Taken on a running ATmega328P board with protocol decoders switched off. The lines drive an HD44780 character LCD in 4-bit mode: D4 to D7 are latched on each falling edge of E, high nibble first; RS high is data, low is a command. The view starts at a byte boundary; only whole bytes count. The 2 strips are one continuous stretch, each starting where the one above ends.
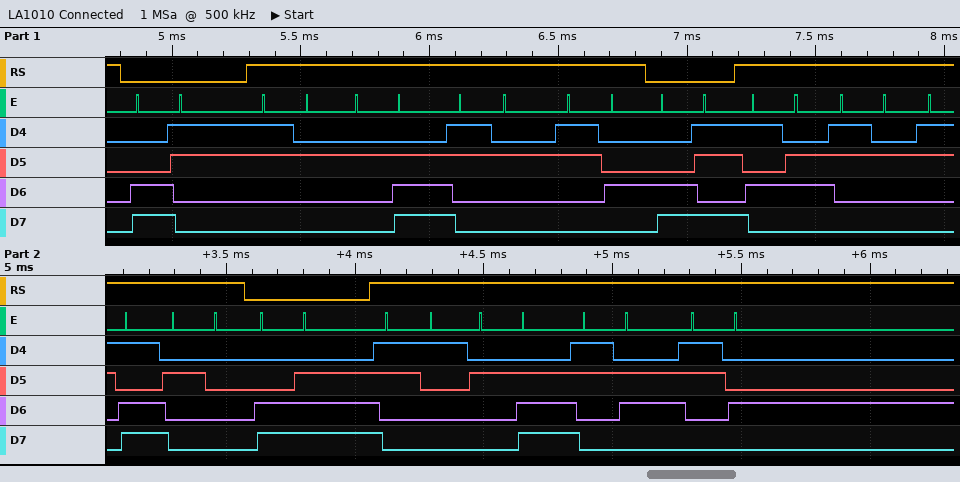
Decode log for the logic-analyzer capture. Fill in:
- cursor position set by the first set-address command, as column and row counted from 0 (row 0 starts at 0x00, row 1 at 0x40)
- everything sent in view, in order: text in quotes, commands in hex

column 3, row 1
0xC3 "2.24" 0xCB "V2= " 0xCE "1.64"
